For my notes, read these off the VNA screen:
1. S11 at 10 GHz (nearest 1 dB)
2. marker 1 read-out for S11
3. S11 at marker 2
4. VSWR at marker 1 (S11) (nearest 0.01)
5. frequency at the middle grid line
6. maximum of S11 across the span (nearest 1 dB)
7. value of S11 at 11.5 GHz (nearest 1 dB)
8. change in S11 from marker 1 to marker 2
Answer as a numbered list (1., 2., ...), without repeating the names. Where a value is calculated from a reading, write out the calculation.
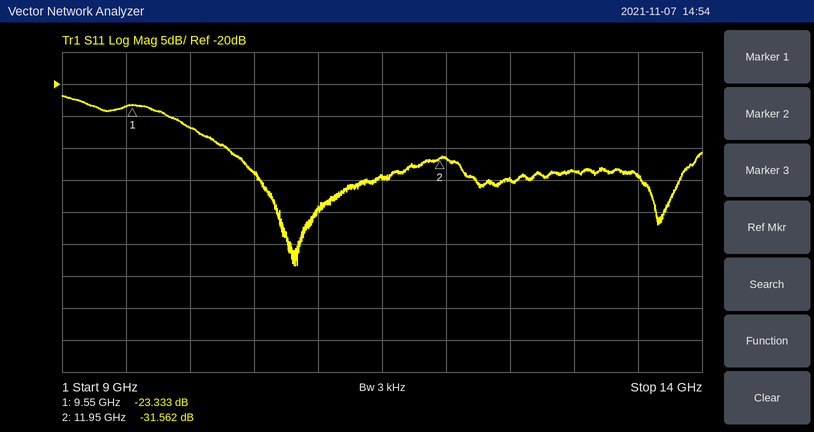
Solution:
1. -27 dB
2. -23.333 dB
3. -31.562 dB
4. (1 + 0.0681)/(1 − 0.0681) ≈ 1.15
5. 11.5 GHz
6. -22 dB
7. -34 dB
8. -31.562 − (-23.333) = -8.229 dB
